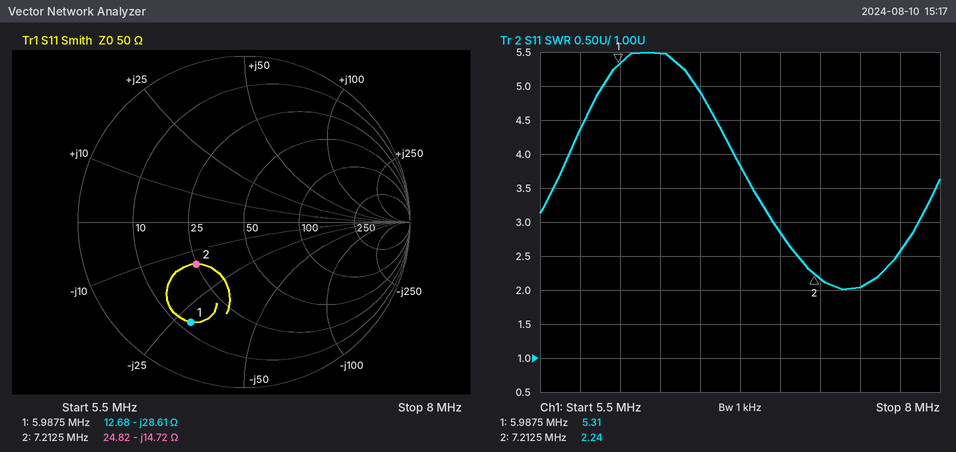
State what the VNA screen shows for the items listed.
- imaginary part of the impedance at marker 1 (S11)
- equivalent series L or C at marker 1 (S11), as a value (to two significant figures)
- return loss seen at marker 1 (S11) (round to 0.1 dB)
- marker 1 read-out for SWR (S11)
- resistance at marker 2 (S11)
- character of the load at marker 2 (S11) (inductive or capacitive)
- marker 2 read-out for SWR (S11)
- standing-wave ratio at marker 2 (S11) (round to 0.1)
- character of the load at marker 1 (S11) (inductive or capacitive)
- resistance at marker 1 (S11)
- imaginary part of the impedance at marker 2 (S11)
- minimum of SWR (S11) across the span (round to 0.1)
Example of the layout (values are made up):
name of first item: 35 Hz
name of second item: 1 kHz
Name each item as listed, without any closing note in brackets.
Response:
imaginary part of the impedance at marker 1: -28.61 Ω
equivalent series L or C at marker 1 (S11), as a value: 930 pF
return loss seen at marker 1 (S11): 3.3 dB
marker 1 read-out for SWR: 5.31
resistance at marker 2: 24.82 Ω
character of the load at marker 2 (S11): capacitive
marker 2 read-out for SWR: 2.24
standing-wave ratio at marker 2 (S11): 2.2
character of the load at marker 1 (S11): capacitive
resistance at marker 1: 12.68 Ω
imaginary part of the impedance at marker 2: -14.72 Ω
minimum of SWR (S11) across the span: 2.0
